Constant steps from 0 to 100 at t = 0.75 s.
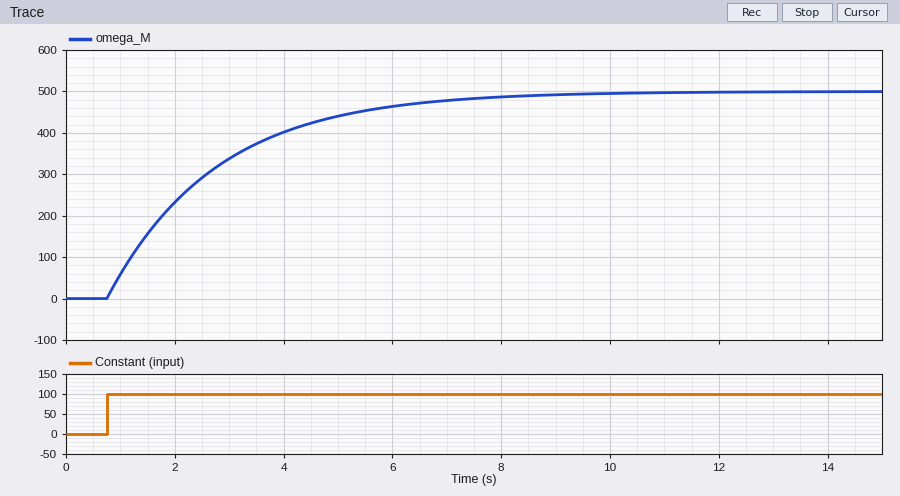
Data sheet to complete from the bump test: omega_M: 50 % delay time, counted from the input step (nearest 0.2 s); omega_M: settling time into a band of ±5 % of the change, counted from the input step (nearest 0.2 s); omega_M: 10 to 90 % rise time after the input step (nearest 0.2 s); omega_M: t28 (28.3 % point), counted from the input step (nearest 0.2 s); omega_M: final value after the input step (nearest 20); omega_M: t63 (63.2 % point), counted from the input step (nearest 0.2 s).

1.4 s
6.0 s
4.4 s
0.6 s
500
2.0 s
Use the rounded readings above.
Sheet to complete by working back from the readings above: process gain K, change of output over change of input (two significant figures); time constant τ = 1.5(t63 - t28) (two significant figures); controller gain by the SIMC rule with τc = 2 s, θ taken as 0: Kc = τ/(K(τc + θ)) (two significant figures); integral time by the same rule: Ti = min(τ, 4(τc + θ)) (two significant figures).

5.0
2.1 s
0.21
2.1 s
